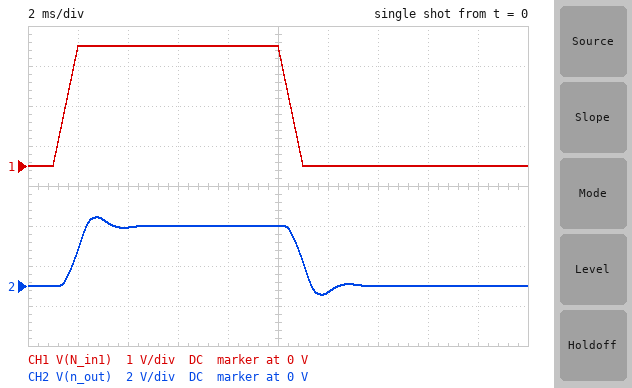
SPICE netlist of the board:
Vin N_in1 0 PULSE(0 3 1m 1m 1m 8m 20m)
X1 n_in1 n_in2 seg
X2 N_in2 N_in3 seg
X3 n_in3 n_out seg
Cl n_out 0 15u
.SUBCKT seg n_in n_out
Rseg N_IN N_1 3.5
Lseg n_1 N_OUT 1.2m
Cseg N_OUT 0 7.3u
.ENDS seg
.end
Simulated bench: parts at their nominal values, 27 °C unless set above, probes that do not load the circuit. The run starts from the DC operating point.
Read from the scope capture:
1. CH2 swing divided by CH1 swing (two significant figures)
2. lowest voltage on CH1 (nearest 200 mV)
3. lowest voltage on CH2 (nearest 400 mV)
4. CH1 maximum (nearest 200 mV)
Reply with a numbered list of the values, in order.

1. 1.3
2. 0 V
3. -400 mV
4. 3.0 V
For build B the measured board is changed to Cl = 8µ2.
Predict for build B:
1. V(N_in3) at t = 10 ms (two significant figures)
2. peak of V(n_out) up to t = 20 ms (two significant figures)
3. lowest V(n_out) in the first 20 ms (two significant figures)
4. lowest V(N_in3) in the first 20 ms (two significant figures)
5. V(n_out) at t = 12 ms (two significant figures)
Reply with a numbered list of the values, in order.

1. 3.0 V
2. 3.5 V
3. -500 mV
4. -400 mV
5. -140 mV
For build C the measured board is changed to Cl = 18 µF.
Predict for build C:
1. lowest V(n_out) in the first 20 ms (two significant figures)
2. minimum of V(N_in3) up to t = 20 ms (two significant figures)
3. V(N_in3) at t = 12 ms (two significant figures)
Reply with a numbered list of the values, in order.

1. -410 mV
2. -310 mV
3. -230 mV
